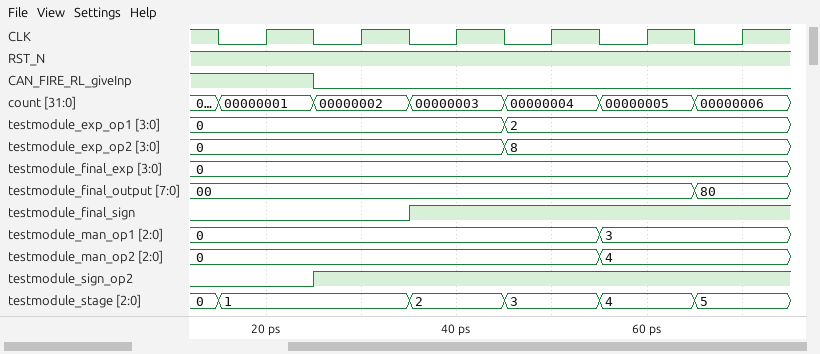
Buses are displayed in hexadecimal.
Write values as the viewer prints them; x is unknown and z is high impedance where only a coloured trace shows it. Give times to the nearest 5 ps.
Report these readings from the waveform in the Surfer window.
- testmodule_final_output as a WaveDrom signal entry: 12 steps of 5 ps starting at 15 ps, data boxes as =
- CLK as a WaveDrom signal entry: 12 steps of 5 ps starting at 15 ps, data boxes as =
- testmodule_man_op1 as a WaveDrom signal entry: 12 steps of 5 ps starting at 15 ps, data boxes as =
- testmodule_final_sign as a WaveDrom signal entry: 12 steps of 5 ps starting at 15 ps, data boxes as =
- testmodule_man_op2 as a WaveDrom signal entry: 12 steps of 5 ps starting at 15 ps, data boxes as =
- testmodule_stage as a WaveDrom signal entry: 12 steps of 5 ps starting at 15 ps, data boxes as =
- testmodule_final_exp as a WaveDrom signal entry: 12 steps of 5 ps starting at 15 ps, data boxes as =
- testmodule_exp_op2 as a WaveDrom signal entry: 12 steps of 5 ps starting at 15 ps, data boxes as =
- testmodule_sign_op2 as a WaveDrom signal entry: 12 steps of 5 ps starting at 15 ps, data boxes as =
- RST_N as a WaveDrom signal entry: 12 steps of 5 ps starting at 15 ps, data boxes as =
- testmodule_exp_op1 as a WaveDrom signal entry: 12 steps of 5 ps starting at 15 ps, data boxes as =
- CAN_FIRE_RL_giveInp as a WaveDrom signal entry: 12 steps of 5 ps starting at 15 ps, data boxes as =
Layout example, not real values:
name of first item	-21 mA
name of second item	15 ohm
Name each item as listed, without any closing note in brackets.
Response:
testmodule_final_output as a WaveDrom signal entry: 12 steps of 5 ps starting at 15 ps, data boxes as =	{name: 'testmodule_final_output', wave: '=.........=.', data: '00 80'}
CLK as a WaveDrom signal entry: 12 steps of 5 ps starting at 15 ps, data boxes as =	{name: 'CLK', wave: '010101010101'}
testmodule_man_op1 as a WaveDrom signal entry: 12 steps of 5 ps starting at 15 ps, data boxes as =	{name: 'testmodule_man_op1', wave: '=.......=...', data: '0 3'}
testmodule_final_sign as a WaveDrom signal entry: 12 steps of 5 ps starting at 15 ps, data boxes as =	{name: 'testmodule_final_sign', wave: '0...1.......'}
testmodule_man_op2 as a WaveDrom signal entry: 12 steps of 5 ps starting at 15 ps, data boxes as =	{name: 'testmodule_man_op2', wave: '=.......=...', data: '0 4'}
testmodule_stage as a WaveDrom signal entry: 12 steps of 5 ps starting at 15 ps, data boxes as =	{name: 'testmodule_stage', wave: '=...=.=.=.=.', data: '1 2 3 4 5'}
testmodule_final_exp as a WaveDrom signal entry: 12 steps of 5 ps starting at 15 ps, data boxes as =	{name: 'testmodule_final_exp', wave: '=...........', data: '0'}
testmodule_exp_op2 as a WaveDrom signal entry: 12 steps of 5 ps starting at 15 ps, data boxes as =	{name: 'testmodule_exp_op2', wave: '=.....=.....', data: '0 8'}
testmodule_sign_op2 as a WaveDrom signal entry: 12 steps of 5 ps starting at 15 ps, data boxes as =	{name: 'testmodule_sign_op2', wave: '0.1.........'}
RST_N as a WaveDrom signal entry: 12 steps of 5 ps starting at 15 ps, data boxes as =	{name: 'RST_N', wave: '1...........'}
testmodule_exp_op1 as a WaveDrom signal entry: 12 steps of 5 ps starting at 15 ps, data boxes as =	{name: 'testmodule_exp_op1', wave: '=.....=.....', data: '0 2'}
CAN_FIRE_RL_giveInp as a WaveDrom signal entry: 12 steps of 5 ps starting at 15 ps, data boxes as =	{name: 'CAN_FIRE_RL_giveInp', wave: '1.0.........'}
